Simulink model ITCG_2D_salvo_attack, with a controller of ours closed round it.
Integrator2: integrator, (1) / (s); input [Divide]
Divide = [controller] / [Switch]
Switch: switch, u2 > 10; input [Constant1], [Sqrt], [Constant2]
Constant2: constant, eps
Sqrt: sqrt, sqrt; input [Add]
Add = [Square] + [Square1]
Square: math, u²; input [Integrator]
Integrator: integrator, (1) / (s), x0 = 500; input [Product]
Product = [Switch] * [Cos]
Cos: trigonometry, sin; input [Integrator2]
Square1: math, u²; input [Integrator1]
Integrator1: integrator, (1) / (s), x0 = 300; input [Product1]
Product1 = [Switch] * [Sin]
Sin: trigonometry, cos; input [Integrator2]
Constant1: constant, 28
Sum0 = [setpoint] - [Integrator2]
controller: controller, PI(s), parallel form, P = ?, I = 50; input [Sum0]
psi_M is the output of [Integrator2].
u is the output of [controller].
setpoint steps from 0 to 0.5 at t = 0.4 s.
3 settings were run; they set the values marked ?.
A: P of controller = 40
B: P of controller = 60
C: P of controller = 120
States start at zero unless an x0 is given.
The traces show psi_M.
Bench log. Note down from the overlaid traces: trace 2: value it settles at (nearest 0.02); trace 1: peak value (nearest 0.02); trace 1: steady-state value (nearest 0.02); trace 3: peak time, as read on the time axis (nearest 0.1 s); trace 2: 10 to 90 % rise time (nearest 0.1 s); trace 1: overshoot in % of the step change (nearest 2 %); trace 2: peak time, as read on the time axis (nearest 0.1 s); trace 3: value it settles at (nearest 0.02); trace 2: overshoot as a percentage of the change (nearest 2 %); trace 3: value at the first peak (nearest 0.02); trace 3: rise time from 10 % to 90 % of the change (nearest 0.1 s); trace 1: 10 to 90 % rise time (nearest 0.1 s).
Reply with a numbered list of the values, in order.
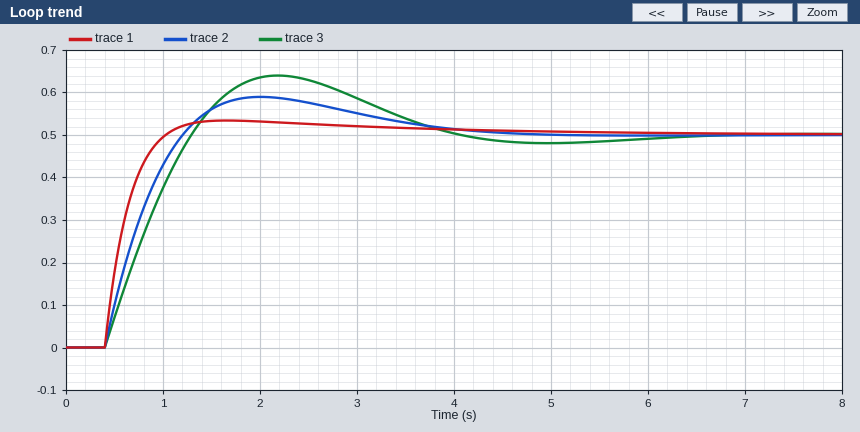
1. 0.50
2. 0.54
3. 0.50
4. 2.2 s
5. 0.6 s
6. 6 %
7. 2.0 s
8. 0.50
9. 18 %
10. 0.64
11. 0.7 s
12. 0.4 s
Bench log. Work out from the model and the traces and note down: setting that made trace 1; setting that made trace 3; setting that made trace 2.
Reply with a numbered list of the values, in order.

1. C
2. A
3. B
